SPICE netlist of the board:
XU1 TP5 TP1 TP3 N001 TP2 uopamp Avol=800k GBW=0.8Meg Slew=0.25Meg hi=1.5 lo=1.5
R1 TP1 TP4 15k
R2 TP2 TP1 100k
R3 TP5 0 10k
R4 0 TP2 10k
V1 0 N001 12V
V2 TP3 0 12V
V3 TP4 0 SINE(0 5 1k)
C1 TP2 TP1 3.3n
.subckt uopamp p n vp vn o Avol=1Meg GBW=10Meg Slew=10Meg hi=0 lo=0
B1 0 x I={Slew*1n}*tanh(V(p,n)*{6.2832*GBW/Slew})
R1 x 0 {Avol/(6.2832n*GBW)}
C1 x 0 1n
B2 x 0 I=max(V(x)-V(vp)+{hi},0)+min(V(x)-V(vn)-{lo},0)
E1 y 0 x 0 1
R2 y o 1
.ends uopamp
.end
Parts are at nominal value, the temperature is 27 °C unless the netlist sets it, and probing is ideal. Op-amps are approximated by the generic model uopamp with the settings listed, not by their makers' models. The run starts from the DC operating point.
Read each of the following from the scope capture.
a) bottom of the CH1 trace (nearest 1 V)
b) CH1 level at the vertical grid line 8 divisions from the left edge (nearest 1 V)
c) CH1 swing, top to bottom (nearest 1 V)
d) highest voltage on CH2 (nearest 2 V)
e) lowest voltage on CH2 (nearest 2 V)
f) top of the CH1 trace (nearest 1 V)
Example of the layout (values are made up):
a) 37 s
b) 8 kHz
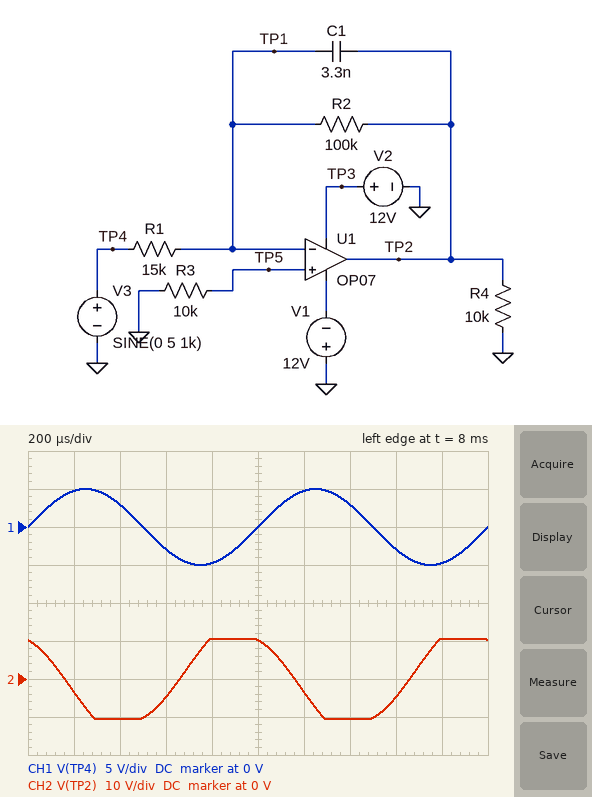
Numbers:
a) -5 V
b) -3 V
c) 10 V
d) 10 V
e) -10 V
f) 5 V
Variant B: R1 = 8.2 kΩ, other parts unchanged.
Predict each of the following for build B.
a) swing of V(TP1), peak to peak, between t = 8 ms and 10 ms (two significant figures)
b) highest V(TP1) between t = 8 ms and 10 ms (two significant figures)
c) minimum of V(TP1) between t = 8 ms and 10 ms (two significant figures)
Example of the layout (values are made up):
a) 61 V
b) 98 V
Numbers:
a) 7.3 V
b) 3.7 V
c) -3.7 V
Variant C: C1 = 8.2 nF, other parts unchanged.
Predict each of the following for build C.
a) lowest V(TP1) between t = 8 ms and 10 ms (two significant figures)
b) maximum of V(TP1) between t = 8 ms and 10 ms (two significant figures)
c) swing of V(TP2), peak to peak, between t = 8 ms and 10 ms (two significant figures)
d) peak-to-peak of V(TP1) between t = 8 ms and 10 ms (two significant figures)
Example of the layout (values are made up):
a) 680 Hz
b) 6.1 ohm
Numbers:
a) -8.0 mV
b) 8.0 mV
c) 13 V
d) 16 mV
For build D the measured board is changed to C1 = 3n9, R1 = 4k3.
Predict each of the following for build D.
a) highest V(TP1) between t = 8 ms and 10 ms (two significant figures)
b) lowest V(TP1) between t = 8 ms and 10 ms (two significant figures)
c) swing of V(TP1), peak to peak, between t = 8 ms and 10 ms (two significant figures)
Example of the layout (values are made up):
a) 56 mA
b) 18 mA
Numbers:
a) 4.3 V
b) -4.3 V
c) 8.7 V
